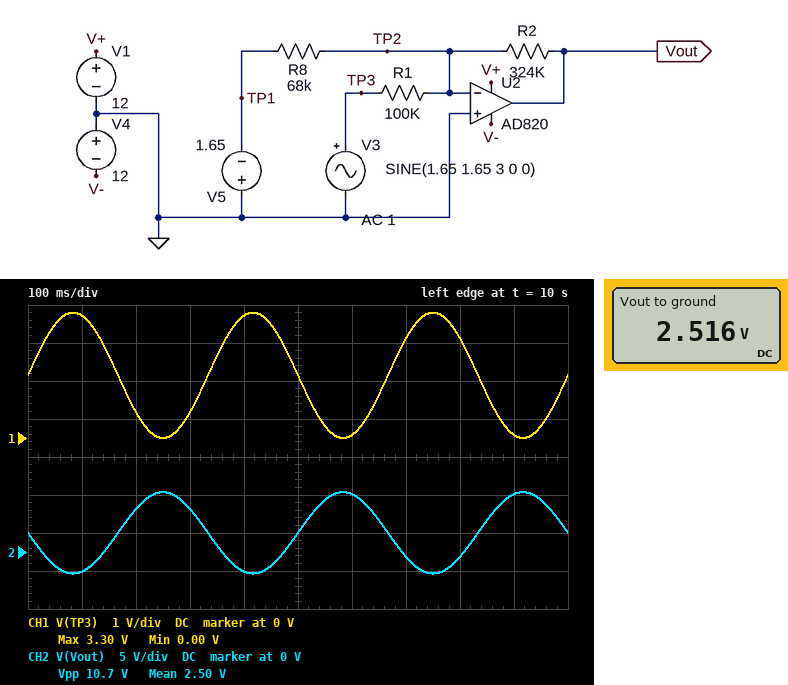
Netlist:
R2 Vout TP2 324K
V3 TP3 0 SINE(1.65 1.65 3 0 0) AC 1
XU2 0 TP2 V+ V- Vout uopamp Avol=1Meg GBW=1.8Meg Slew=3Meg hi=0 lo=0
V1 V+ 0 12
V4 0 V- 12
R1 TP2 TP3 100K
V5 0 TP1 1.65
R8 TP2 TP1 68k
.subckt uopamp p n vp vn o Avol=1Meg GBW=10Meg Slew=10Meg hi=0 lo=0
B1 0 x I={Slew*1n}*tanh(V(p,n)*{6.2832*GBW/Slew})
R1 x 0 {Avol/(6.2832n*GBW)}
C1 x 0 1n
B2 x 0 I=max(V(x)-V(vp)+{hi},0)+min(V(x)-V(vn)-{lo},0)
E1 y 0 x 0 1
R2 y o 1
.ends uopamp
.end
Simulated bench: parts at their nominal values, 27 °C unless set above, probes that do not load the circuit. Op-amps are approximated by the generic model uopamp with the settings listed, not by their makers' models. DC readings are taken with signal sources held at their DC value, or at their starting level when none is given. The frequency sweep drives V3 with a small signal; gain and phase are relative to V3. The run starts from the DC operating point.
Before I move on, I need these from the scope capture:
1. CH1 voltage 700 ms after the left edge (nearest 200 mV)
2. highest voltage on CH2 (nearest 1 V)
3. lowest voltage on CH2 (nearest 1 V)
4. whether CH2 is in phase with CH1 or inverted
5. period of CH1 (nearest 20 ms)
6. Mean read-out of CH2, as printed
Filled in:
2.6 V
8 V
-3 V
inverted
340 ms
2.50 V
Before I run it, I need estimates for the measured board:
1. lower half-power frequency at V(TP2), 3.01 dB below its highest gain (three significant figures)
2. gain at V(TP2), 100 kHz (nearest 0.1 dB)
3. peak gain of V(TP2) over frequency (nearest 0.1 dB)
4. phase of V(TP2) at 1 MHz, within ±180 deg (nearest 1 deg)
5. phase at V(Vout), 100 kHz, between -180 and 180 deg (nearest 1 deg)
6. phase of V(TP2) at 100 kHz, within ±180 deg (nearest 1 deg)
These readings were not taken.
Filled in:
200 kHz
-15.9 dB
-8.9 dB
11 deg
153 deg
63 deg
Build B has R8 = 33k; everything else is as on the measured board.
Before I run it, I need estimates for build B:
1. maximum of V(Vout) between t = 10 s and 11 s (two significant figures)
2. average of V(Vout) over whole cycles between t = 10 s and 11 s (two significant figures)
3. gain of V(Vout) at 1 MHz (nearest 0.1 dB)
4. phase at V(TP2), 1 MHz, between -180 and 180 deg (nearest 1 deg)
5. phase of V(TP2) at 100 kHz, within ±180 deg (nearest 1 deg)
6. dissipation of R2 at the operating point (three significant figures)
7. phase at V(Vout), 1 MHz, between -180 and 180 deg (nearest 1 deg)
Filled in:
12 V
9.7 V
-7.7 dB
7 deg
52 deg
364 µW
97 deg
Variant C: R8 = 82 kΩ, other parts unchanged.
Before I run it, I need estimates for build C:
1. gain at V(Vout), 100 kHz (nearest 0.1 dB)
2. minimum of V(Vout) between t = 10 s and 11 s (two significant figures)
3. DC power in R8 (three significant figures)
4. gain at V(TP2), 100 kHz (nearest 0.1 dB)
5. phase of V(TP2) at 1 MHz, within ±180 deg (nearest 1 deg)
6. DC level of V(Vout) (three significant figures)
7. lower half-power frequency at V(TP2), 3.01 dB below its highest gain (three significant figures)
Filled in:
9.4 dB
-4.2 V
33.2 µW
-15.7 dB
12 deg
1.17 V
220 kHz
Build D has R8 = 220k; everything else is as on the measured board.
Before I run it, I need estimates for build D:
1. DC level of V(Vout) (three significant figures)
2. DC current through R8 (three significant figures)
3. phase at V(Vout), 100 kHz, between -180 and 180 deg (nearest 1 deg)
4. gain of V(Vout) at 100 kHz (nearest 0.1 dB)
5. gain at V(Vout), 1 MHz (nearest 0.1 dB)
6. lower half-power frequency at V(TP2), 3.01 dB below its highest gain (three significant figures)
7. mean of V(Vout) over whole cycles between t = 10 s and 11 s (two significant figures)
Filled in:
-2.92 V
7.50 µA
162 deg
9.8 dB
-0.2 dB
315 kHz
-2.9 V
